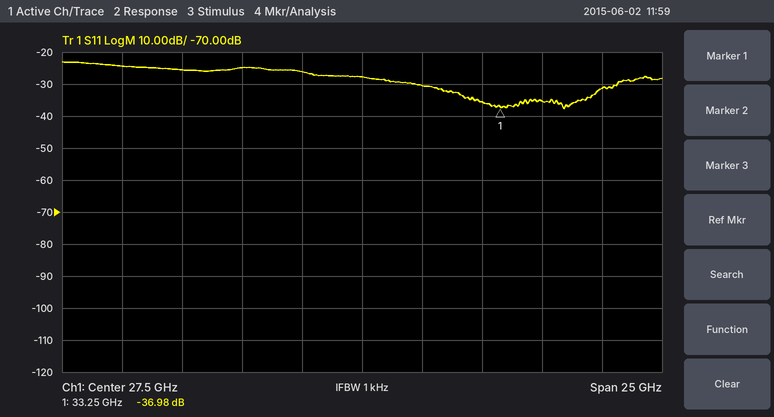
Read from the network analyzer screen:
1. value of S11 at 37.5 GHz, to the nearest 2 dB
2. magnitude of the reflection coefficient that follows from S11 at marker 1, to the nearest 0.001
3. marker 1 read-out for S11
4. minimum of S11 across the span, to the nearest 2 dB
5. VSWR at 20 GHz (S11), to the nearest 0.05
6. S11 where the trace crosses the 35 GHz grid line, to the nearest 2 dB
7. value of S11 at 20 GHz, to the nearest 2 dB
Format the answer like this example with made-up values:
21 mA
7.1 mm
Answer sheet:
-32 dB
0.014
-36.98 dB
-38 dB
1.10
-36 dB
-26 dB
